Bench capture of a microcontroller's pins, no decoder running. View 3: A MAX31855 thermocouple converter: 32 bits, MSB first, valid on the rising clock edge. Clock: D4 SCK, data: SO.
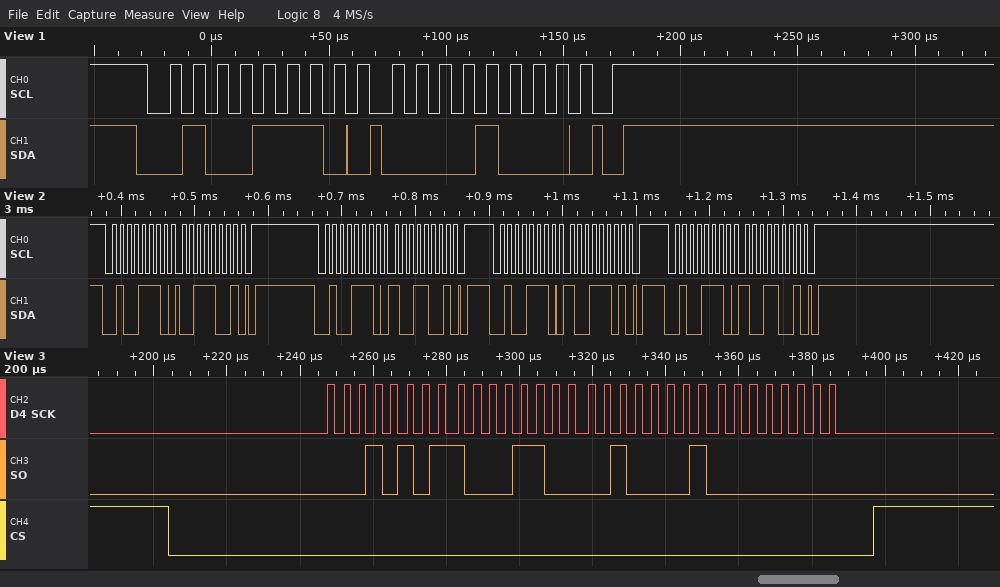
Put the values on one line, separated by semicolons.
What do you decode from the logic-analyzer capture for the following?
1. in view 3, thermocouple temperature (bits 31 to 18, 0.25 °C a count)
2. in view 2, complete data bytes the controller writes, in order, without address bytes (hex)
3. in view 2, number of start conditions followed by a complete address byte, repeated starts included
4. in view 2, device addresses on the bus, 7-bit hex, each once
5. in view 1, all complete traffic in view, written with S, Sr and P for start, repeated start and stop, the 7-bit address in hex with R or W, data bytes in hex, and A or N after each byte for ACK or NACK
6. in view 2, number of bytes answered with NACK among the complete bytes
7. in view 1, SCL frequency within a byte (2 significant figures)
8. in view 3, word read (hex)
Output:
344.75 °C; 39 99 9D 99; 4; 0x27; S 27W A 08 A P; 0; 100 kHz; 0x158C2100
